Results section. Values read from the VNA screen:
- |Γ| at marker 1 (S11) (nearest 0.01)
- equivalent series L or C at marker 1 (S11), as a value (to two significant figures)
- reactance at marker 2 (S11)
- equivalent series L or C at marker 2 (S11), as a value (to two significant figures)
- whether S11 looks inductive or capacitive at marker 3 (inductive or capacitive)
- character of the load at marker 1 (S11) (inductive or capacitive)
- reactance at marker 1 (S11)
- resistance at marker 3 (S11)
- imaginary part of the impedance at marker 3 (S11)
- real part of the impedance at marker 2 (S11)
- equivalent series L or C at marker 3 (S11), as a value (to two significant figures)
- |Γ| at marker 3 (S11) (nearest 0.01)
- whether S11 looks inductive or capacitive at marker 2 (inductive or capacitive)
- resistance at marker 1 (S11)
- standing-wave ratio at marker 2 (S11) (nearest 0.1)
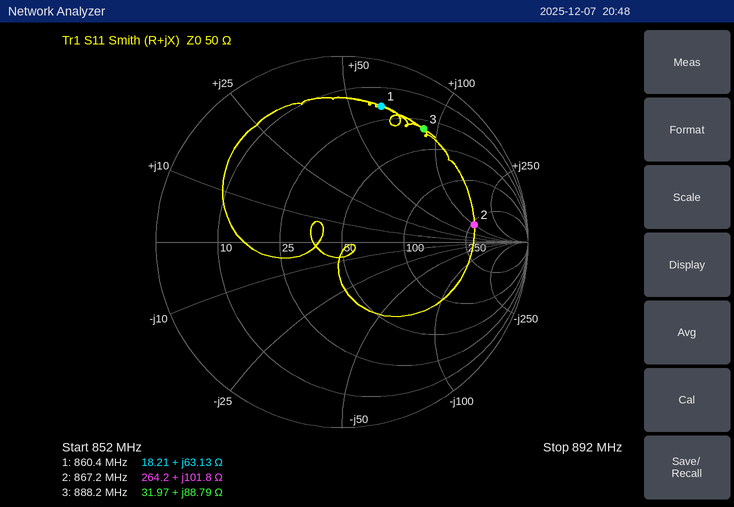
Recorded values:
0.76
12 nH
+101.8 Ω
19 nH
inductive
inductive
+63.13 Ω
31.97 Ω
+88.79 Ω
264.2 Ω
16 nH
0.75
inductive
18.21 Ω
6.1
